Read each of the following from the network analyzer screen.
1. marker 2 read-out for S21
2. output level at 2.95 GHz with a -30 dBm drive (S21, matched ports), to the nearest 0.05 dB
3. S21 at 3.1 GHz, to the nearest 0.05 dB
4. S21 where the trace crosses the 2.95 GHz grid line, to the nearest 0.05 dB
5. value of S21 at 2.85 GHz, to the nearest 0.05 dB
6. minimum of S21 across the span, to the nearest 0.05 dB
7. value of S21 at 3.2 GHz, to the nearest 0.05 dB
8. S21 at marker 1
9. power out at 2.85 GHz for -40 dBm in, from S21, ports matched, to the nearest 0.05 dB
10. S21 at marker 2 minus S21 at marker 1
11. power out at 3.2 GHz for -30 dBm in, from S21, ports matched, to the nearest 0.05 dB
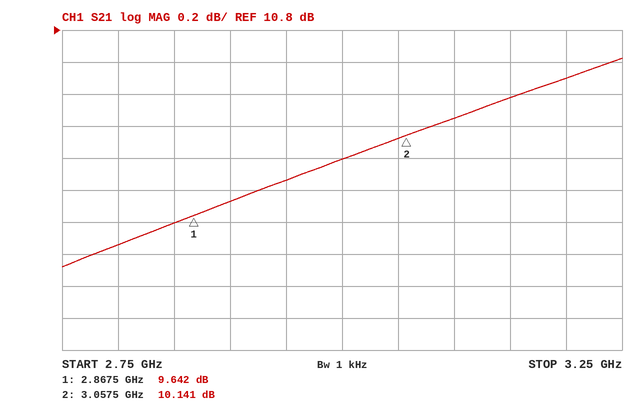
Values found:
10.141 dB
-20.15 dBm
10.25 dB
9.85 dB
9.60 dB
9.30 dB
10.50 dB
9.642 dB
-30.40 dBm
0.499 dB
-19.50 dBm
